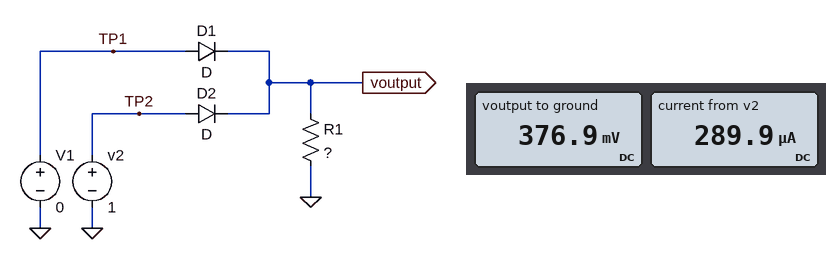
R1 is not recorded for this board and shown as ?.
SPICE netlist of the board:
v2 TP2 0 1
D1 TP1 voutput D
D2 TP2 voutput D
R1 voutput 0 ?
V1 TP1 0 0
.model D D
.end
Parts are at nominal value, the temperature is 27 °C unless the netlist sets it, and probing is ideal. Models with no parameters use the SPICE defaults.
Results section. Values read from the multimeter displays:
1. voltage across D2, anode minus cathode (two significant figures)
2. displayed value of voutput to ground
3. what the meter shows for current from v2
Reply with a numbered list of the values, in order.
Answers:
1. 620 mV
2. 376.9 mV
3. 289.9 µA
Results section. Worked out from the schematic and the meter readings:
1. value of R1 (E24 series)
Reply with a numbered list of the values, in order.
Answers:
1. 1.3 kΩ
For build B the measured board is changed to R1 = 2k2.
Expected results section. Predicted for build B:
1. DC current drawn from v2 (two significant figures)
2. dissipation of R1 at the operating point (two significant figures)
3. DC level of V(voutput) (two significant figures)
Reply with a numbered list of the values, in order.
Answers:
1. 180 µA
2. 69 µW
3. 390 mV
